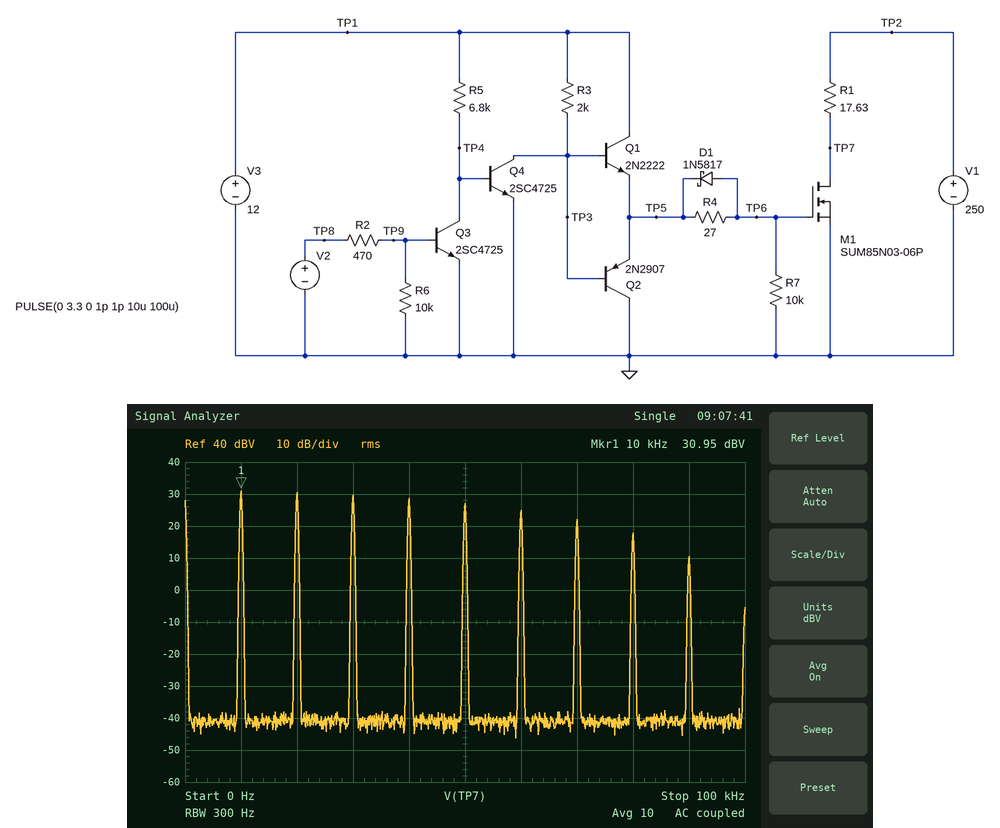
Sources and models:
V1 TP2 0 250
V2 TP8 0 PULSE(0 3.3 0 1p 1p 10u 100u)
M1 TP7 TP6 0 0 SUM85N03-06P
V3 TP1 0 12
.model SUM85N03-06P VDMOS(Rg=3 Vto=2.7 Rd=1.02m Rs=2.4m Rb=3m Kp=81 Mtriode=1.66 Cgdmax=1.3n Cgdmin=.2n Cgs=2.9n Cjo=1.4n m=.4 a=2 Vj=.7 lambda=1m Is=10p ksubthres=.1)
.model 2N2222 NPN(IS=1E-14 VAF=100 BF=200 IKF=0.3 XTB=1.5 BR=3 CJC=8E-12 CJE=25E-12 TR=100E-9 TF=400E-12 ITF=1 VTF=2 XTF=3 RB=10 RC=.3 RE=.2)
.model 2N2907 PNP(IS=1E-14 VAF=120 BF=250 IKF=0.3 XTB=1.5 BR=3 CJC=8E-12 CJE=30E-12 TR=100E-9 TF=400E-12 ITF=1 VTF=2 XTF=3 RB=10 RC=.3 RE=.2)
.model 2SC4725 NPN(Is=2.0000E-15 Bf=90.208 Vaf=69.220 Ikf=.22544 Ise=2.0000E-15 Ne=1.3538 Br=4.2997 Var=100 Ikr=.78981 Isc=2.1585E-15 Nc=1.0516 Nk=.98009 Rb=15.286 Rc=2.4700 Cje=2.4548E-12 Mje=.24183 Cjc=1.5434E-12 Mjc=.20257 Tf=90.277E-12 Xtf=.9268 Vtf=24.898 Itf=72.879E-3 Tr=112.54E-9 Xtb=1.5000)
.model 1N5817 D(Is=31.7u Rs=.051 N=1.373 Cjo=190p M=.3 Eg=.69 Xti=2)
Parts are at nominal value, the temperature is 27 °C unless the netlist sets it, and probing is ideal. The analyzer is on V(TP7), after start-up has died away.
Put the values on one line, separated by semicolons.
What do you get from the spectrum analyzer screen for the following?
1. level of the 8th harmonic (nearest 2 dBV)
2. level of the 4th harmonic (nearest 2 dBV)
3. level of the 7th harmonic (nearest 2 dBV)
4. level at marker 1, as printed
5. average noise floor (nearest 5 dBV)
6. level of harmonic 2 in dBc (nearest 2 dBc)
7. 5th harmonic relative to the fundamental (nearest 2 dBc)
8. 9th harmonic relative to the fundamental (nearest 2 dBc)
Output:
18 dBV; 28 dBV; 22 dBV; 30.95 dBV; -40 dBV; 0 dBc; -4 dBc; -20 dBc
